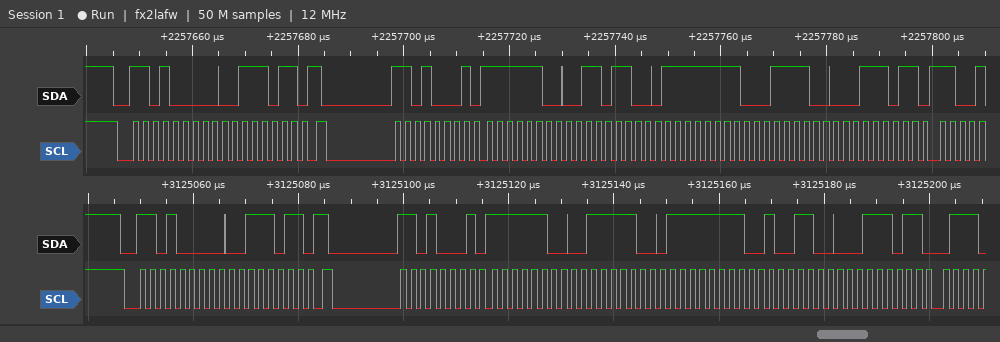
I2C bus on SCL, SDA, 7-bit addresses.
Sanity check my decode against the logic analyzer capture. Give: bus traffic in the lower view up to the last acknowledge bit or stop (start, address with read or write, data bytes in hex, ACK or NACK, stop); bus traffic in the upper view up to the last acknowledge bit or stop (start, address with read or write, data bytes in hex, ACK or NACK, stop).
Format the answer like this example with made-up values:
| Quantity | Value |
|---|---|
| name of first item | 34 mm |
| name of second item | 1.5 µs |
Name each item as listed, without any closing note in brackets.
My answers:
| Quantity | Value |
|---|---|
| bus traffic in the lower view up to the last acknowledge bit or stop | start, address 68 write ACK, 3B ACK, repeated start, address 68 read ACK, FC ACK, 7C ACK, FF ACK, 4C ACK, 3B ACK |
| bus traffic in the upper view up to the last acknowledge bit or stop | start, address 68 write ACK, 3B ACK, repeated start, address 68 read ACK, FC ACK, 6C ACK, FF ACK, 3C ACK, 3B ACK |
